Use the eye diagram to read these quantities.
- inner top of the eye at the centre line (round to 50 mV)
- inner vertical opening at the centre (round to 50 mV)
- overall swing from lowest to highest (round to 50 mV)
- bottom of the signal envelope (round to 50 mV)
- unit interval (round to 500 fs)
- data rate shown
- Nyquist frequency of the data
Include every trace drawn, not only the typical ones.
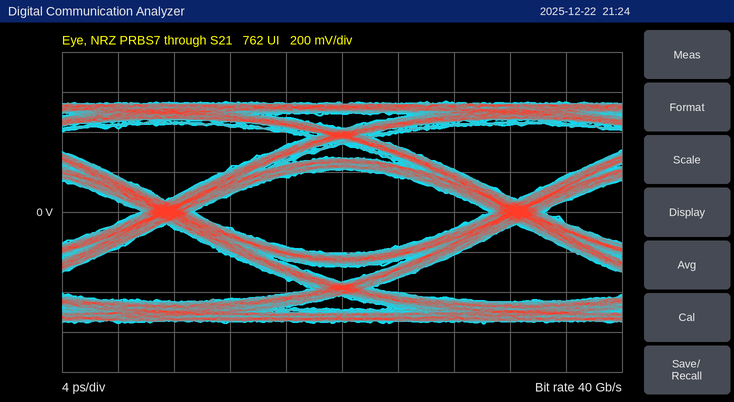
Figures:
200 mV
400 mV
1.10 V
-550 mV
25.0 ps
40 Gb/s
20 GHz
